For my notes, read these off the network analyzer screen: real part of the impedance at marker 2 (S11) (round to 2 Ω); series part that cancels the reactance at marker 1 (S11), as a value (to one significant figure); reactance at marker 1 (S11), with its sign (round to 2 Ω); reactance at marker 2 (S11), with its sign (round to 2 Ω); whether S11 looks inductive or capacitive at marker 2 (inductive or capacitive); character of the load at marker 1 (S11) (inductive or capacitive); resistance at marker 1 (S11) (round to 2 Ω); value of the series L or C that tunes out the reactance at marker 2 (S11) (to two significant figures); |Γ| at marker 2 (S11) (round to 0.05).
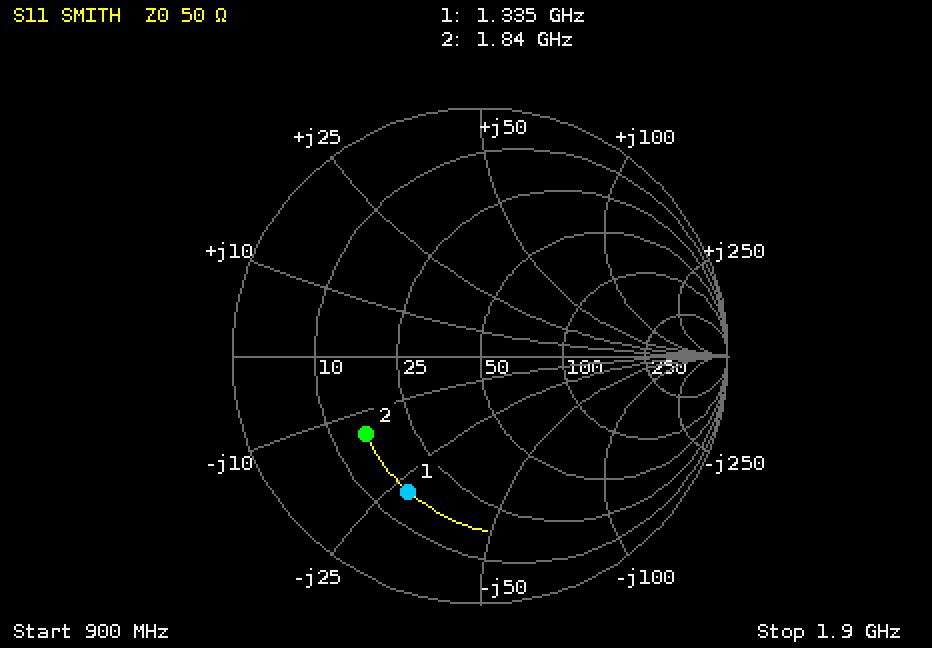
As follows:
16 Ω
3 nH
-28 Ω
-14 Ω
capacitive
capacitive
16 Ω
1.2 nH
0.55
